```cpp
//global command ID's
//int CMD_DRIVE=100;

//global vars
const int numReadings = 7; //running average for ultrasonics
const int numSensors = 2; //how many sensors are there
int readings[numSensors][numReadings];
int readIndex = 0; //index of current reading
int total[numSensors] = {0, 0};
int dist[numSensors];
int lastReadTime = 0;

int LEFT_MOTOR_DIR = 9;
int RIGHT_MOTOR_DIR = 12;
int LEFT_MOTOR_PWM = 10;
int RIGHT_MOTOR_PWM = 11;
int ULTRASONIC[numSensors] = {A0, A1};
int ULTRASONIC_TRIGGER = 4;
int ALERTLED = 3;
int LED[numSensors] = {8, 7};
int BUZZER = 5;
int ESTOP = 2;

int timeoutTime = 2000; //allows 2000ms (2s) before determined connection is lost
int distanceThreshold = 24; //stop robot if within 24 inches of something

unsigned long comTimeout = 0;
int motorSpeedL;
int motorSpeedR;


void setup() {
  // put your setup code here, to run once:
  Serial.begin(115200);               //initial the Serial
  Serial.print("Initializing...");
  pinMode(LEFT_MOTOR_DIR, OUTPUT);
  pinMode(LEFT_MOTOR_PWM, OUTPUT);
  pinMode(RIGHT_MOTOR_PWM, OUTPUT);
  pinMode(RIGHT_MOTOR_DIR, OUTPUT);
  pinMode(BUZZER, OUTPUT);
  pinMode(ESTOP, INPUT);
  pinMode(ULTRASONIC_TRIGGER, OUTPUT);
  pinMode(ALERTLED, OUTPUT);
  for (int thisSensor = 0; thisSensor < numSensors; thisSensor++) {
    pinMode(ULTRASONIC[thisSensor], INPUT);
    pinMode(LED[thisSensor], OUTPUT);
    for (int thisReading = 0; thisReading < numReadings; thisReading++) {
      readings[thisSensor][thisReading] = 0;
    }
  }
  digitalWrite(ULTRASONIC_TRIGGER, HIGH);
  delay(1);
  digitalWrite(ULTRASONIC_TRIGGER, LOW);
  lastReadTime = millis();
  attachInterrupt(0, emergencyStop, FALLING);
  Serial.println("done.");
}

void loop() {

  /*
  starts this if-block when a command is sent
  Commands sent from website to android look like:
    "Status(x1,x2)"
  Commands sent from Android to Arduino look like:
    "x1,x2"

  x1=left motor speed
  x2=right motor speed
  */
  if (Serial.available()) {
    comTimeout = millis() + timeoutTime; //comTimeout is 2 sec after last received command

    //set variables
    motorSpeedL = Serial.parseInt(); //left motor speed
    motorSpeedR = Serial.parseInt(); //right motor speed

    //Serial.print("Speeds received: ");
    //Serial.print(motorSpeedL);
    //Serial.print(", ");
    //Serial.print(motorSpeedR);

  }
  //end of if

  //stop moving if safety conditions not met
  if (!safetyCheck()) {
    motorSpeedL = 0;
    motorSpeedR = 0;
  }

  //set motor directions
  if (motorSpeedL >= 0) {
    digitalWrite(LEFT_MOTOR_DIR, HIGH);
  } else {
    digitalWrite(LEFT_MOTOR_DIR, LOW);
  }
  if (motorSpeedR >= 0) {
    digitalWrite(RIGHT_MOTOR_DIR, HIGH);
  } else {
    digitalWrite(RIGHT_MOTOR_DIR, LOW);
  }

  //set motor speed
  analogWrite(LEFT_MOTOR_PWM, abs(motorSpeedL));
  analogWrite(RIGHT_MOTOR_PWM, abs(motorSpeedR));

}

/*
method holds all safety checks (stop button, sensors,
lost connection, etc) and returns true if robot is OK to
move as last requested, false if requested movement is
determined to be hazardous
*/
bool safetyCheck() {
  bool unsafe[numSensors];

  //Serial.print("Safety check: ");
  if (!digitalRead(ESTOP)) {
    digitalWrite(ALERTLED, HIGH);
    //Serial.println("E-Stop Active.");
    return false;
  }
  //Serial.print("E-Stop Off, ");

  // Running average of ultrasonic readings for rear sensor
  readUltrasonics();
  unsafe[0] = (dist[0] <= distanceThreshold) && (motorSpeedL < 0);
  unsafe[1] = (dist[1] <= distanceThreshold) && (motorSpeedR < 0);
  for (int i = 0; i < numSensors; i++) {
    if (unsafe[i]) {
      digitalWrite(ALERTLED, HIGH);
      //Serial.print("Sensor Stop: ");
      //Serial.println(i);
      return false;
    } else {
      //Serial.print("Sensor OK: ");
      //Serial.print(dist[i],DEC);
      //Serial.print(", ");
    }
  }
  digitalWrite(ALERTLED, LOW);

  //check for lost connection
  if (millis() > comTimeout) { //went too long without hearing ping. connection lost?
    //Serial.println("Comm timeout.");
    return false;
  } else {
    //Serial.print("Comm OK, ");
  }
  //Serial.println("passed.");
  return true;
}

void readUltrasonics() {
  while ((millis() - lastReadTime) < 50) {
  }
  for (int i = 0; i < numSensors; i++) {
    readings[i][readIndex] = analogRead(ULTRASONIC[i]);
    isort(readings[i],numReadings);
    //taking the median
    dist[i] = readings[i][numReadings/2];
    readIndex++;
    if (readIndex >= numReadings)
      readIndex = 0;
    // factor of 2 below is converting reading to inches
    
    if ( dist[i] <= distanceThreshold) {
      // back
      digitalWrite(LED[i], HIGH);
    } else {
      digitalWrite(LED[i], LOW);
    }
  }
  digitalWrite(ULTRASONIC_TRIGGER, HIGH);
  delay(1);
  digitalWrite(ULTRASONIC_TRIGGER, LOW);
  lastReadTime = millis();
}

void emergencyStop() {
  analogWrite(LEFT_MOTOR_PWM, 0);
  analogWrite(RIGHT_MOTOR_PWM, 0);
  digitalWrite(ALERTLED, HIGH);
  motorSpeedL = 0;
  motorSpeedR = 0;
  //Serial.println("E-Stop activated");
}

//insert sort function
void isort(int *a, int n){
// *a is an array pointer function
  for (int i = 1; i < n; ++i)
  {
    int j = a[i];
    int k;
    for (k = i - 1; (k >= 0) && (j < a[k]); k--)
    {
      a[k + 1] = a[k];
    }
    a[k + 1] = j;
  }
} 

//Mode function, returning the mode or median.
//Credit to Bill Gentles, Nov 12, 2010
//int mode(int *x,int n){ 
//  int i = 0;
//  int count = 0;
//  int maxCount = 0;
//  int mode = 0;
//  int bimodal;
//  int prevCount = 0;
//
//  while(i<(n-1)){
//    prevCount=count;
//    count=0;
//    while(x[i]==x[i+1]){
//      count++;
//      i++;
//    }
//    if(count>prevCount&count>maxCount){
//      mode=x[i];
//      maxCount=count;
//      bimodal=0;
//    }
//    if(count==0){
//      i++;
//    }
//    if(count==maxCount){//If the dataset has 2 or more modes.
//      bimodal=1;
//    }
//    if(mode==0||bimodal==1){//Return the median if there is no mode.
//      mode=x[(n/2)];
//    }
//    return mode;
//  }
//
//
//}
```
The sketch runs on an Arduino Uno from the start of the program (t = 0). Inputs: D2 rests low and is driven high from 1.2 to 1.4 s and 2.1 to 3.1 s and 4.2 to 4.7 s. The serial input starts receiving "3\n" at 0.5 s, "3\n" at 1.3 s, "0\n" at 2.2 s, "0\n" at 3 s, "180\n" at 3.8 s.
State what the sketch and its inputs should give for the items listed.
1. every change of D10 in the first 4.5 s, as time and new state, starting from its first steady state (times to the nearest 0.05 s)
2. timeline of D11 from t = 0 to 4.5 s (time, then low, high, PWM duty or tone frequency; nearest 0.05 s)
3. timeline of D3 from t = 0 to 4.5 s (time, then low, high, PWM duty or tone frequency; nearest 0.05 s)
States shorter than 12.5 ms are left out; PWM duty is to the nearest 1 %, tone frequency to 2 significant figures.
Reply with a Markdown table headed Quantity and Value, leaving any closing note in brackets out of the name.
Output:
| Quantity | Value |
|---|---|
| every change of D10 in the first 4.5 s, as time and new state, starting from its first steady state | 0 s low; 1.3 s PWM 1 %; 1.4 s low |
| timeline of D11 from t = 0 to 4.5 s | 0 s low; 1.3 s PWM 1 %; 1.4 s low |
| timeline of D3 from t = 0 to 4.5 s | 0 s high; 1.3 s low; 1.4 s high; 3 s low; 3.1 s high |
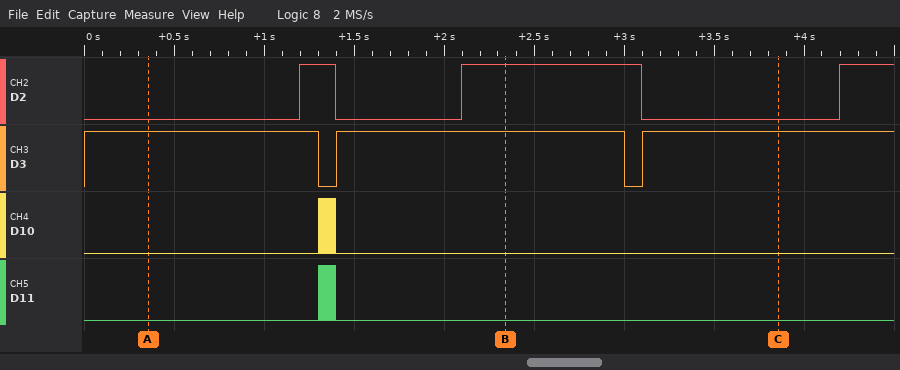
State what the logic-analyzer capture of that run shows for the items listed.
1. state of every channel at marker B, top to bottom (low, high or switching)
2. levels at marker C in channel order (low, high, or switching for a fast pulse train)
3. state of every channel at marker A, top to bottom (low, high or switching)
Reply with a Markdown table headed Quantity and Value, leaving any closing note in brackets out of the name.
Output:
| Quantity | Value |
|---|---|
| state of every channel at marker B, top to bottom | D2 high, D3 high, D10 low, D11 low |
| levels at marker C in channel order | D2 low, D3 high, D10 low, D11 low |
| state of every channel at marker A, top to bottom | D2 low, D3 high, D10 low, D11 low |
